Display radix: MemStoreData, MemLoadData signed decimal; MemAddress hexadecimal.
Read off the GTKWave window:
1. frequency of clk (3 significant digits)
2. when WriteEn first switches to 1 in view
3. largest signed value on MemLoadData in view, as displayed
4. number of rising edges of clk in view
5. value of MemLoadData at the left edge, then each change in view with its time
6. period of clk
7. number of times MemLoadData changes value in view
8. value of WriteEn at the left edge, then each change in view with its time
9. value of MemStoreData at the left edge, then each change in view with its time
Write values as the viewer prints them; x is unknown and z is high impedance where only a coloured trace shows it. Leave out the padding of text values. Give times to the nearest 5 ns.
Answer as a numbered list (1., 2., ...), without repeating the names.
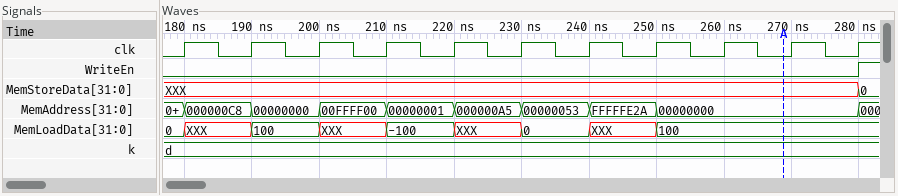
1. 100 MHz
2. 280 ns
3. 100
4. 11
5. 0, XXX at 180 ns, 100 at 190 ns, XXX at 200 ns, -100 at 210 ns, XXX at 220 ns, 0 at 230 ns, XXX at 240 ns, 100 at 250 ns
6. 10 ns
7. 8
8. 0, 1 at 280 ns
9. XXX, 0 at 280 ns
